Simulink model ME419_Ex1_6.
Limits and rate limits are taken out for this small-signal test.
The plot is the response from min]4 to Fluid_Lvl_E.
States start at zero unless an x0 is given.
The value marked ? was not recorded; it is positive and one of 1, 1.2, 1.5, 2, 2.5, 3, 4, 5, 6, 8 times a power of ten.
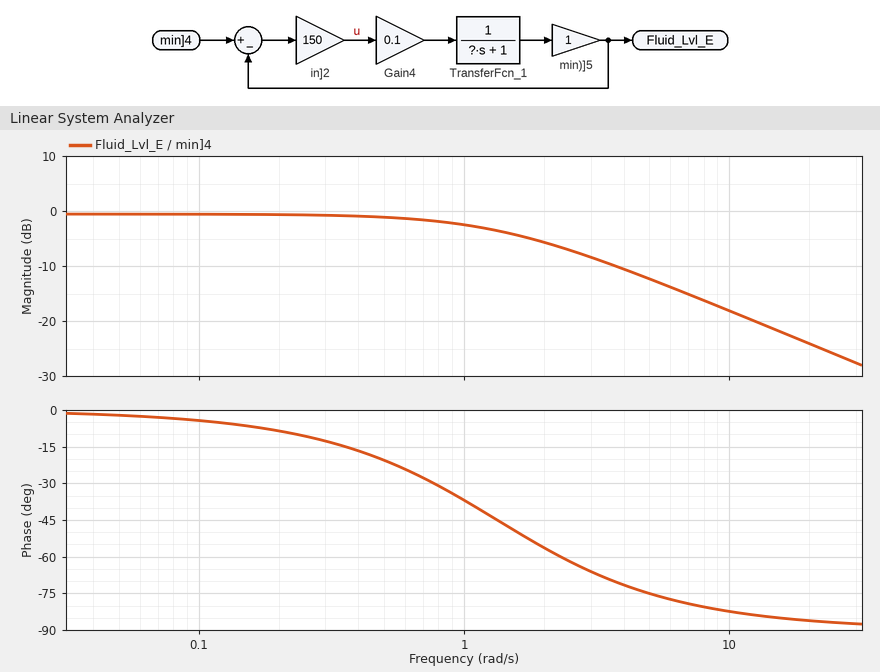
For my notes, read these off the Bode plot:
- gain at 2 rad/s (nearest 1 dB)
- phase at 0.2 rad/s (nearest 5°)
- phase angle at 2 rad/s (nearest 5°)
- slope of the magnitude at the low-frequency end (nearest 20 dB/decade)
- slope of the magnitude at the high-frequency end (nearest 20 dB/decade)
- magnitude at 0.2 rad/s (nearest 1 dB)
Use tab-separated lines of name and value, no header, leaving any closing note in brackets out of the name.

gain at 2 rad/s	-6 dB
phase at 0.2 rad/s	-10°
phase angle at 2 rad/s	-55°
slope of the magnitude at the low-frequency end	0 dB/decade
slope of the magnitude at the high-frequency end	-20 dB/decade
magnitude at 0.2 rad/s	-1 dB
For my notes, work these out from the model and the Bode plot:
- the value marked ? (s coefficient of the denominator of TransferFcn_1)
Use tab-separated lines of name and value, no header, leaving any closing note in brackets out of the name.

the value marked ?	12
